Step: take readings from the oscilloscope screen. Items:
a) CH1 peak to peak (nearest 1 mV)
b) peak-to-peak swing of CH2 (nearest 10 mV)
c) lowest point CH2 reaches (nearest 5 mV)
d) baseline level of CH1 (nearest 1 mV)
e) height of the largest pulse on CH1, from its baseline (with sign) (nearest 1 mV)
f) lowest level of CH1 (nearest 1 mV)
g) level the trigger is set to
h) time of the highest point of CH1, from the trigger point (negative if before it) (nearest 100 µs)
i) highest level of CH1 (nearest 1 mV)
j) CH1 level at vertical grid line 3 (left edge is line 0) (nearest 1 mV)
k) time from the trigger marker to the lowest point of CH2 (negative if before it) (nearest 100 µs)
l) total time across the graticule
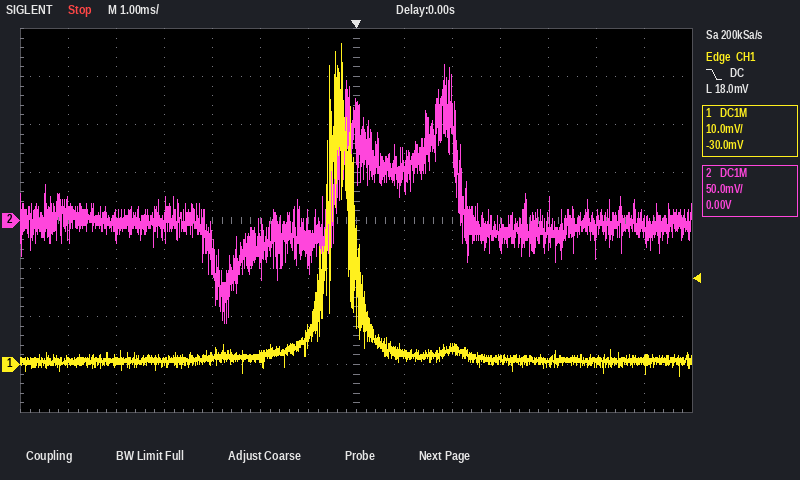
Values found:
69 mV
270 mV
-105 mV
1 mV
+66 mV
-2 mV
18.0 mV
-300 µs
67 mV
1 mV
-2.7 ms
14 ms
